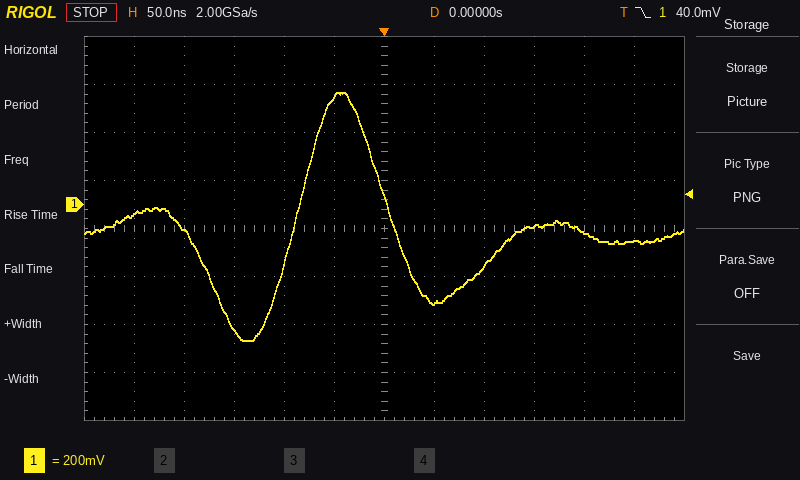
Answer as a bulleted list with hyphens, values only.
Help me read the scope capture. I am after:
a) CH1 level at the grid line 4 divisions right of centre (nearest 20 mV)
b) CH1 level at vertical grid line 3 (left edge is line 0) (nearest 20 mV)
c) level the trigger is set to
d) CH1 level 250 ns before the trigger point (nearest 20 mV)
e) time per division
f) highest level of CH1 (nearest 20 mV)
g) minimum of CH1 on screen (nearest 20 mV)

- -120 mV
- -520 mV
- 40.0 mV
- -40 mV
- 50 ns
- 460 mV
- -560 mV
